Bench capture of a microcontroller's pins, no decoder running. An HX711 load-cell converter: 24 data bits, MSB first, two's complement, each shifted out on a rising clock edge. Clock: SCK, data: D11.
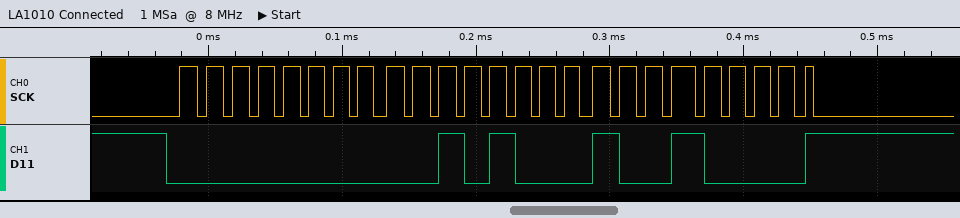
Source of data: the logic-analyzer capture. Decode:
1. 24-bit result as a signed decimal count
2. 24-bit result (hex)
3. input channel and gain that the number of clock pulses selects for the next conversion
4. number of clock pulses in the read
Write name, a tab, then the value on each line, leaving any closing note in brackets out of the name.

24-bit result as a signed decimal count	10384
24-bit result	0x002890
input channel and gain that the number of clock pulses selects for the next conversion	channel A, gain 128
number of clock pulses in the read	25
